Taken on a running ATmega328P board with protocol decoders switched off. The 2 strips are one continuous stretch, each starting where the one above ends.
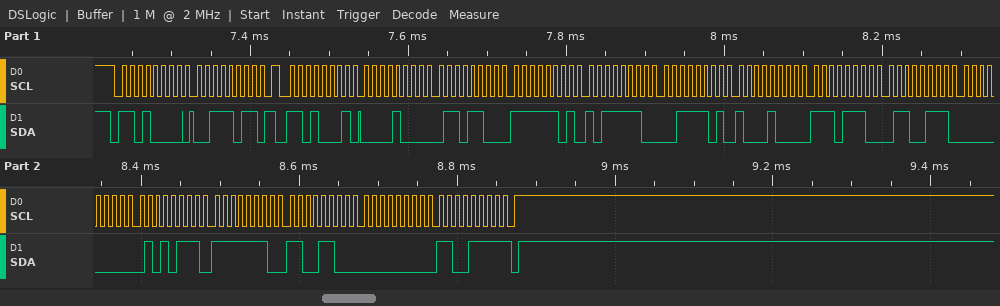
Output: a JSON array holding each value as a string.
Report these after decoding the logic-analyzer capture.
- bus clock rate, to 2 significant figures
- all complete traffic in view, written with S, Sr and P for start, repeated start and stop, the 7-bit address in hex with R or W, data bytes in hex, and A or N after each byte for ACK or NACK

["100 kHz", "S 68W A 3B A Sr 68R A 08 A 6C A FD A BE A 3D A 88 A EE A 67 A 00 A 57 A FE A CC A 00 A CF N P"]
